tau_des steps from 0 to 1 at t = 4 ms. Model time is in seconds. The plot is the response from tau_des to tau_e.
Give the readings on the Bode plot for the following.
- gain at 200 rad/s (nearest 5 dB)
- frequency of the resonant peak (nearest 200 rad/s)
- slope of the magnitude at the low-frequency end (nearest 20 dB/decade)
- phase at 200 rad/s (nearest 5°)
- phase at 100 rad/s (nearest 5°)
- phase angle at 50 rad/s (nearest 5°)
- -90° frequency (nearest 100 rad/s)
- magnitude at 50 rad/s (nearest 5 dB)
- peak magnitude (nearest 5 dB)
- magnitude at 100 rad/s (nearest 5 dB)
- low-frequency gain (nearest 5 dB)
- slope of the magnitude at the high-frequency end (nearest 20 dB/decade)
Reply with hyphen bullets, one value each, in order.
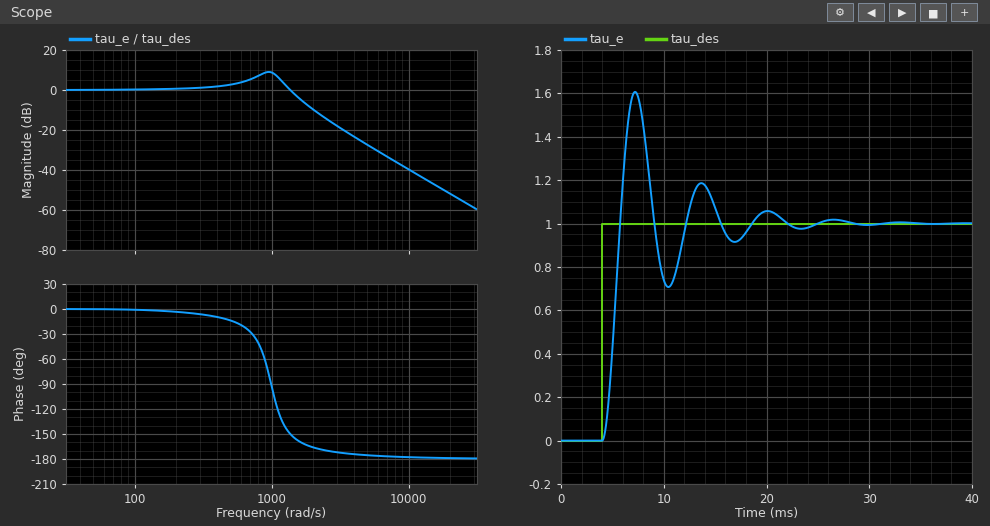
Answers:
- 0 dB
- 1000 rad/s
- 0 dB/decade
- -5°
- 0°
- 0°
- 1000 rad/s
- 0 dB
- 10 dB
- 0 dB
- 0 dB
- -40 dB/decade
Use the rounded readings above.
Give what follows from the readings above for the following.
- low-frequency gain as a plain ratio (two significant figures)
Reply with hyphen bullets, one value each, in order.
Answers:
- 1.0
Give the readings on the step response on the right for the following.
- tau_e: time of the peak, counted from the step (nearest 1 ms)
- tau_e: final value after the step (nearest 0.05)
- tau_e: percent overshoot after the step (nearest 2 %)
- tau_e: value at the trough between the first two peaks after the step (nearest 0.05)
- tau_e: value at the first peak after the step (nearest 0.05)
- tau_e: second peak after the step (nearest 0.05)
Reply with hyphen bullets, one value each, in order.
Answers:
- 3 ms
- 1.00
- 60 %
- 0.70
- 1.60
- 1.20
